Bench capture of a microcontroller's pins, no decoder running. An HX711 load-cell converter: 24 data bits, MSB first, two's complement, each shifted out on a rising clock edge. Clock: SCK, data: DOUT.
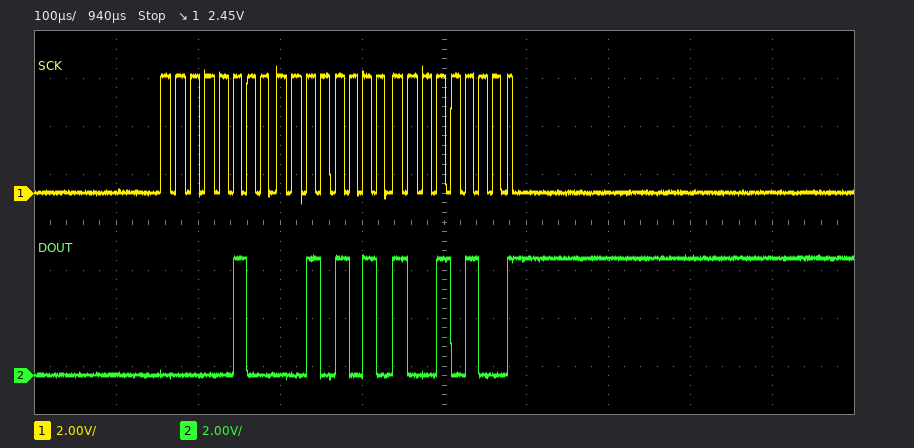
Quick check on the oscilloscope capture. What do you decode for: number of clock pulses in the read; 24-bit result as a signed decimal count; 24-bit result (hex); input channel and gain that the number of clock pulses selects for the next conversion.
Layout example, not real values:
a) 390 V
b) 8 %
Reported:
a) 25
b) 273044
c) 0x042A94
d) channel A, gain 128
